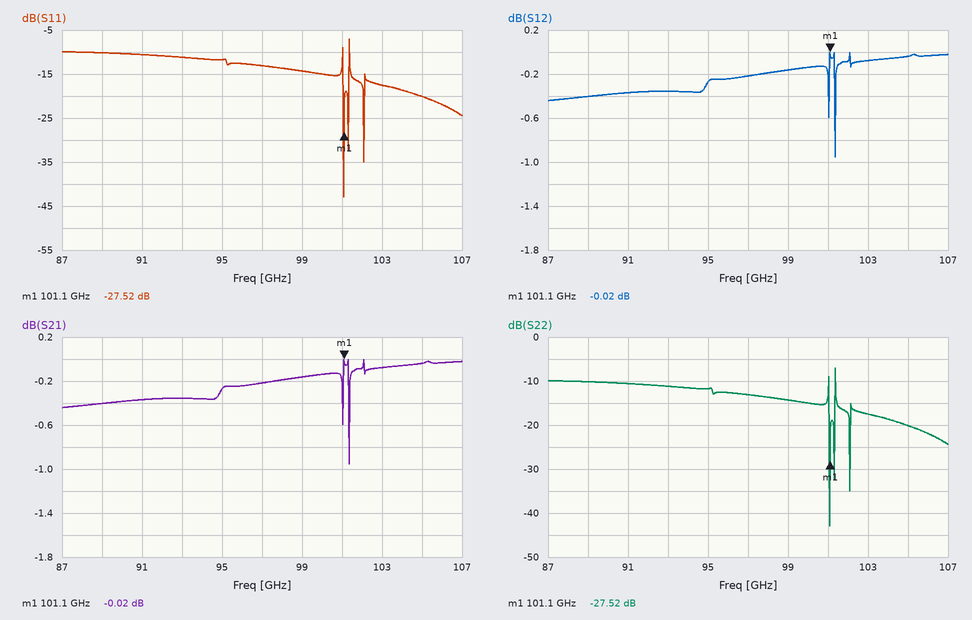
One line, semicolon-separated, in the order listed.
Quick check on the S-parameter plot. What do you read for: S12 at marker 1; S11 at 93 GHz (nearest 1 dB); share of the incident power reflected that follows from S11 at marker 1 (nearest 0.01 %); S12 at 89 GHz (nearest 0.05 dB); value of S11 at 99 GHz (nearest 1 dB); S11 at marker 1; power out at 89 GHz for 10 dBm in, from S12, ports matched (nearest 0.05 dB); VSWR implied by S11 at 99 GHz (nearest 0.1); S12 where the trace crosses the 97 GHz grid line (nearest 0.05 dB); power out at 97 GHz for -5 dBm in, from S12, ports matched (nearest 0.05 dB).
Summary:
-0.02 dB; -11 dB; 0.18 %; -0.40 dB; -14 dB; -27.52 dB; 9.60 dBm; 1.5; -0.20 dB; -5.20 dBm
